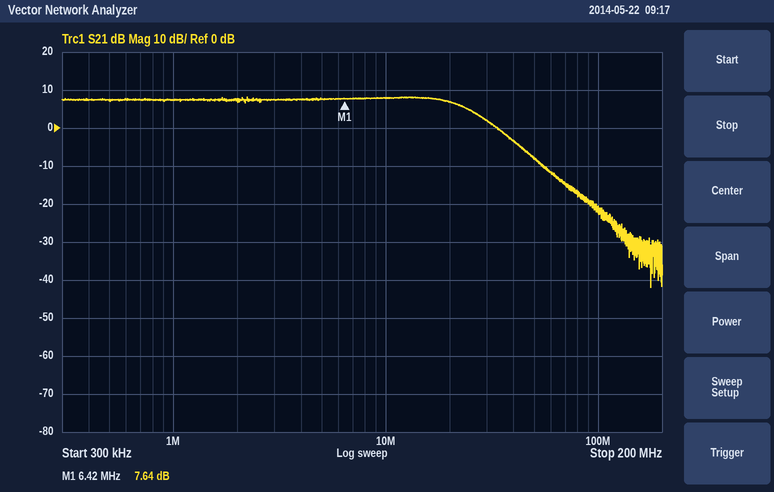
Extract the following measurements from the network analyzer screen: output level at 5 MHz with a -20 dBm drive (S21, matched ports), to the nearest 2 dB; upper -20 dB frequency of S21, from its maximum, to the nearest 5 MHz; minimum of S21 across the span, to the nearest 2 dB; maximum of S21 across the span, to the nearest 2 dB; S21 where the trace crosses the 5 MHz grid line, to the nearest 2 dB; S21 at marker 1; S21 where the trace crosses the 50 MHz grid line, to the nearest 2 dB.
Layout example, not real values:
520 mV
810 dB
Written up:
-12 dBm
60 MHz
-42 dB
8 dB
8 dB
7.64 dB
-8 dB
